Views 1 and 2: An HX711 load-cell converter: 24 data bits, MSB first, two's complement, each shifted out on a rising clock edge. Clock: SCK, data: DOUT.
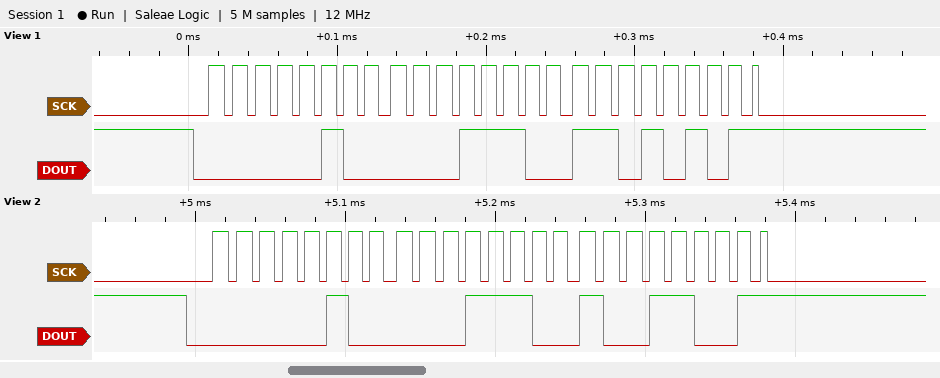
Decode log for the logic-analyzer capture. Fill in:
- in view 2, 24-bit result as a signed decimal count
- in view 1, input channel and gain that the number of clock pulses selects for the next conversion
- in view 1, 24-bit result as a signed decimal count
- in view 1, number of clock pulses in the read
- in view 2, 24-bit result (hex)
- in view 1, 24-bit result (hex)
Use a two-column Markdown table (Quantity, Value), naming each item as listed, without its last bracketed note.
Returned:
| Quantity | Value |
|---|---|
| in view 2, 24-bit result as a signed decimal count | 269465 |
| in view 1, input channel and gain that the number of clock pulses selects for the next conversion | channel A, gain 128 |
| in view 1, 24-bit result as a signed decimal count | 269525 |
| in view 1, number of clock pulses in the read | 25 |
| in view 2, 24-bit result | 0x041C99 |
| in view 1, 24-bit result | 0x041CD5 |
